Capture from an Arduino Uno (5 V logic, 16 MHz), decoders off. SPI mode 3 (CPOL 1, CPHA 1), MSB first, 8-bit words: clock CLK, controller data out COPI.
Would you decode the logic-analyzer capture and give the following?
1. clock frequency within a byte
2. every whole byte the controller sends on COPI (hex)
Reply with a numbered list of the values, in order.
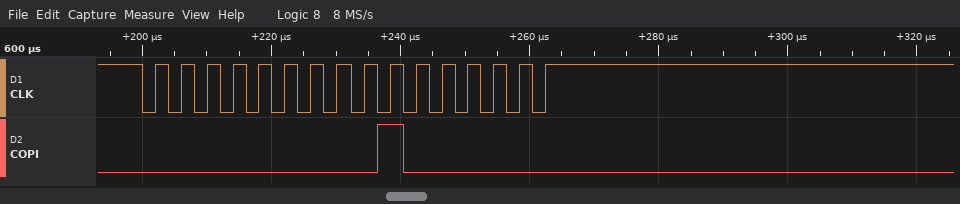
1. 250 kHz
2. 0x00 0x40
